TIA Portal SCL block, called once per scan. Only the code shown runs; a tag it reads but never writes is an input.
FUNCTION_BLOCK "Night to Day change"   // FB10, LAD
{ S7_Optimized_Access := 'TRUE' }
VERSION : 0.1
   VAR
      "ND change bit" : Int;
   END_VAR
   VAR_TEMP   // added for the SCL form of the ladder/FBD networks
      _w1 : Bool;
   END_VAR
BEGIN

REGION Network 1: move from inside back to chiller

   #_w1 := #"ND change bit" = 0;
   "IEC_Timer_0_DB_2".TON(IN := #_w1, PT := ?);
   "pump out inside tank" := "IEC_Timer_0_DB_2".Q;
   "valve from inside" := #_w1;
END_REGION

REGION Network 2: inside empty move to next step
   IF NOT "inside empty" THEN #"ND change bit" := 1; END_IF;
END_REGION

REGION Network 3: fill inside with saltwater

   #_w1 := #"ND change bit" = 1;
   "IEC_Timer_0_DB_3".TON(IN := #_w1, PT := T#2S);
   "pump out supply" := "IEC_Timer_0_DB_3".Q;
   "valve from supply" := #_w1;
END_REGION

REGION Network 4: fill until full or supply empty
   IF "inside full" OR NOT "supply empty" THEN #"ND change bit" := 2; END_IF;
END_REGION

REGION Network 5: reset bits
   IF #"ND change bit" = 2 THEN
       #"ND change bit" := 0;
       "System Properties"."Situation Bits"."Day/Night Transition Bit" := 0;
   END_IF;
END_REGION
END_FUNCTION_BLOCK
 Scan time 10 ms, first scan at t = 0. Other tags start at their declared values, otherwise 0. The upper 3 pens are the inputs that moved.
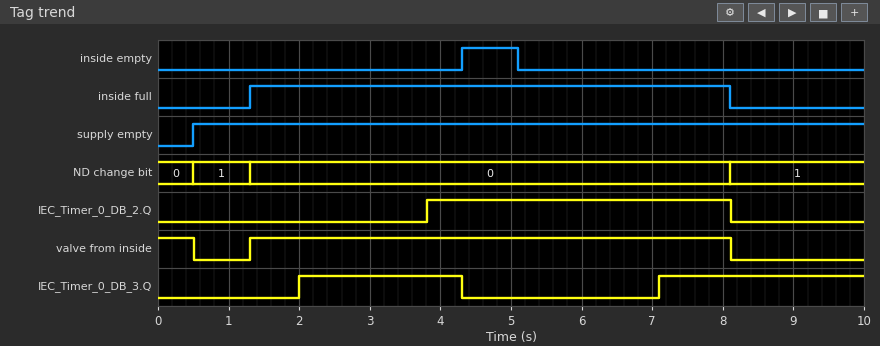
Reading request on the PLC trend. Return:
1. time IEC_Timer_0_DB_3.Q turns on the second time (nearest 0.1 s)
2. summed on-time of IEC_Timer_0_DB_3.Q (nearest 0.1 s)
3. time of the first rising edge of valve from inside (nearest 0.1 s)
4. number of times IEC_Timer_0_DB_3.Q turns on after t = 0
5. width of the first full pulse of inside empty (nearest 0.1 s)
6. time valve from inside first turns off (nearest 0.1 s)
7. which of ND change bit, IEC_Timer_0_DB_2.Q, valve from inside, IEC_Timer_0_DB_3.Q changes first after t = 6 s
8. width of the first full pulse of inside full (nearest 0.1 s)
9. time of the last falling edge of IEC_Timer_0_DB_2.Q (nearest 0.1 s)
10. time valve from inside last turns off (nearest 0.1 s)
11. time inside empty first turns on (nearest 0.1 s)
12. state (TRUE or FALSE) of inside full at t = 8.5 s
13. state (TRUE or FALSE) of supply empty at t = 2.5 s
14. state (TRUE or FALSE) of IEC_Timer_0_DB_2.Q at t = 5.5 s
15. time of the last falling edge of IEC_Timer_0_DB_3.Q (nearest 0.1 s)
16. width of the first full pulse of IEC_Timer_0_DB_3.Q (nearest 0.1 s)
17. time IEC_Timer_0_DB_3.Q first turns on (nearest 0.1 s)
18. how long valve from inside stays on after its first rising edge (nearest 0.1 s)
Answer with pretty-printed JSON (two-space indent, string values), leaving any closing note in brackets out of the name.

{
  "time IEC_Timer_0_DB_3.Q turns on the second time": "7.1 s",
  "summed on-time of IEC_Timer_0_DB_3.Q": "5.2 s",
  "time of the first rising edge of valve from inside": "1.3 s",
  "number of times IEC_Timer_0_DB_3.Q turns on after t = 0": "2",
  "width of the first full pulse of inside empty": "0.8 s",
  "time valve from inside first turns off": "0.5 s",
  "which of ND change bit, IEC_Timer_0_DB_2.Q, valve from inside, IEC_Timer_0_DB_3.Q changes first after t = 6 s": "IEC_Timer_0_DB_3.Q",
  "width of the first full pulse of inside full": "6.8 s",
  "time of the last falling edge of IEC_Timer_0_DB_2.Q": "8.1 s",
  "time valve from inside last turns off": "8.1 s",
  "time inside empty first turns on": "4.3 s",
  "state (TRUE or FALSE) of inside full at t = 8.5 s": "FALSE",
  "state (TRUE or FALSE) of supply empty at t = 2.5 s": "TRUE",
  "state (TRUE or FALSE) of IEC_Timer_0_DB_2.Q at t = 5.5 s": "TRUE",
  "time of the last falling edge of IEC_Timer_0_DB_3.Q": "4.3 s",
  "width of the first full pulse of IEC_Timer_0_DB_3.Q": "2.3 s",
  "time IEC_Timer_0_DB_3.Q first turns on": "2.0 s",
  "how long valve from inside stays on after its first rising edge": "6.8 s"
}
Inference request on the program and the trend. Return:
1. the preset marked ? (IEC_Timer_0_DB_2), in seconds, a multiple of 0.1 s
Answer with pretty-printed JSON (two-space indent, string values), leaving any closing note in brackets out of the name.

{
  "the preset marked ? (IEC_Timer_0_DB_2), in seconds, a multiple of 0.1 s": "2.5 s"
}
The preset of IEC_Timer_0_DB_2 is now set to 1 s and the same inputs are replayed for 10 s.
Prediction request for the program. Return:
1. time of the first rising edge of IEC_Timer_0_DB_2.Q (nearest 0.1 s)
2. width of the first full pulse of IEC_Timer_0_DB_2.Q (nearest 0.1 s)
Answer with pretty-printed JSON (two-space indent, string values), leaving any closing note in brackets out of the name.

{
  "time of the first rising edge of IEC_Timer_0_DB_2.Q": "2.3 s",
  "width of the first full pulse of IEC_Timer_0_DB_2.Q": "5.8 s"
}
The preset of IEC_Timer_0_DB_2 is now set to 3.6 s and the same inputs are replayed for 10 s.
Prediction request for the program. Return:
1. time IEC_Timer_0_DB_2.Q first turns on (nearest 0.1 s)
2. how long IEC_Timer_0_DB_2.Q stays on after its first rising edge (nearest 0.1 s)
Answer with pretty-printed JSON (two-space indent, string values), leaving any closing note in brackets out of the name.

{
  "time IEC_Timer_0_DB_2.Q first turns on": "4.9 s",
  "how long IEC_Timer_0_DB_2.Q stays on after its first rising edge": "3.2 s"
}
